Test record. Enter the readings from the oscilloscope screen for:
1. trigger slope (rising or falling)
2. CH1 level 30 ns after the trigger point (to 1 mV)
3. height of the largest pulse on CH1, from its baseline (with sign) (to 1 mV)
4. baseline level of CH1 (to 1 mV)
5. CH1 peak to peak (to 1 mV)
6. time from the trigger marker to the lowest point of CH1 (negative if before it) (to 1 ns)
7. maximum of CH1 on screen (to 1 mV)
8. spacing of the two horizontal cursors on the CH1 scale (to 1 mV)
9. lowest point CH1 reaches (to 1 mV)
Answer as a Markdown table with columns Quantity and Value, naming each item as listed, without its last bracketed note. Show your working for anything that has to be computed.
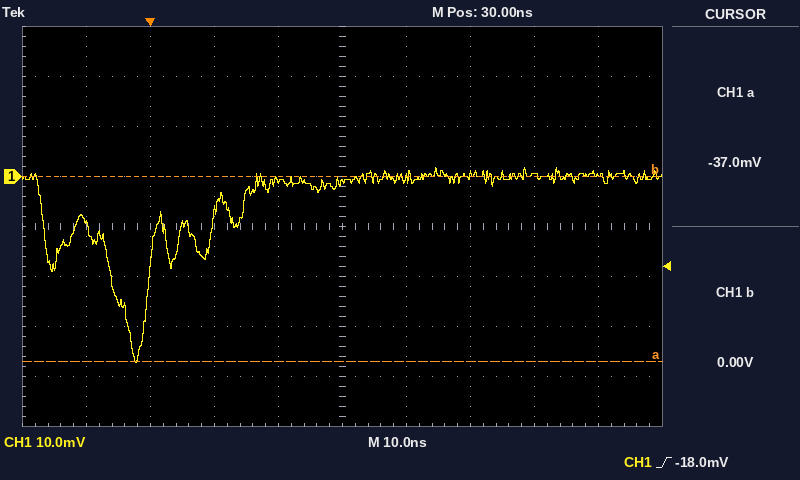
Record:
| Quantity | Value |
|---|---|
| trigger slope | rising |
| CH1 level 30 ns after the trigger point | -1 mV |
| height of the largest pulse on CH1, from its baseline (with sign) | -37 mV − (0 mV) = -37 mV |
| baseline level of CH1 | 0 mV |
| CH1 peak to peak | 2 mV − (-37 mV) = 39 mV |
| time from the trigger marker to the lowest point of CH1 (negative if before it) | -2 ns |
| maximum of CH1 on screen | 2 mV |
| spacing of the two horizontal cursors on the CH1 scale | 37 mV |
| lowest point CH1 reaches | -37 mV |
